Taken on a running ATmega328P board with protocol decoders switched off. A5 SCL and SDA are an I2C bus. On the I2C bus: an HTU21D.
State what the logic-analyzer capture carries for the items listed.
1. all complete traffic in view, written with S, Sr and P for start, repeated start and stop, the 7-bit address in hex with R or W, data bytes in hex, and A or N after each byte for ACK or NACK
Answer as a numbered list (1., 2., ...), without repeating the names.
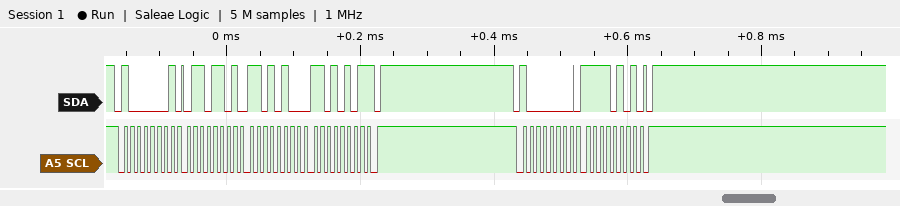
1. S 40R A 6D A D4 A D5 N P S 40W A F5 A P
